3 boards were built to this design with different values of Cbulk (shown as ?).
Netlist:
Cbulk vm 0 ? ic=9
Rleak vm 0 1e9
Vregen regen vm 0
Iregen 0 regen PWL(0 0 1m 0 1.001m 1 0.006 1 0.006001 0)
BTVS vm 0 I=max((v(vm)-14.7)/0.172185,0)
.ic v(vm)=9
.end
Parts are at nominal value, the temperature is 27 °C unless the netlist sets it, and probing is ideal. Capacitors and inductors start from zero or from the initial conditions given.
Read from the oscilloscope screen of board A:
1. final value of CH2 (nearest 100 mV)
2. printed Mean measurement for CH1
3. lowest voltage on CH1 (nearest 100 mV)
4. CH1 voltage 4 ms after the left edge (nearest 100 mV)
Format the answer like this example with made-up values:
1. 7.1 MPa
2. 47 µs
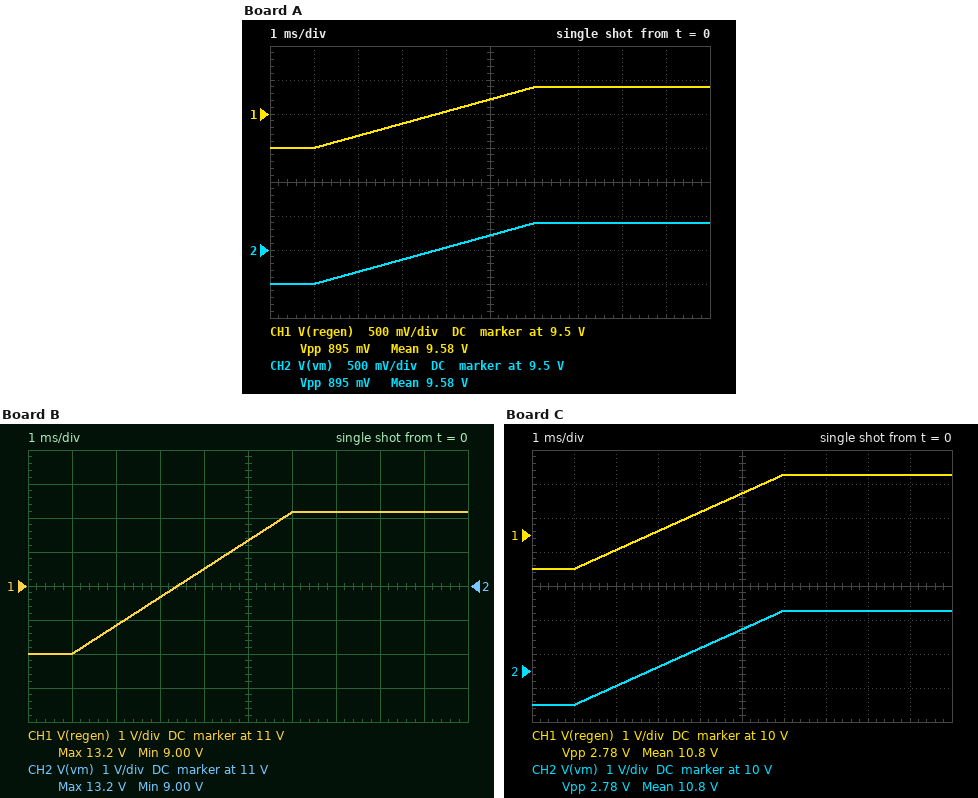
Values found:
1. 9.9 V
2. 9.58 V
3. 9.0 V
4. 9.5 V
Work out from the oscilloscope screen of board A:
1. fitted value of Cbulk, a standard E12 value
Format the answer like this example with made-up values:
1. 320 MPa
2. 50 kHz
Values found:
1. 5.6 mF
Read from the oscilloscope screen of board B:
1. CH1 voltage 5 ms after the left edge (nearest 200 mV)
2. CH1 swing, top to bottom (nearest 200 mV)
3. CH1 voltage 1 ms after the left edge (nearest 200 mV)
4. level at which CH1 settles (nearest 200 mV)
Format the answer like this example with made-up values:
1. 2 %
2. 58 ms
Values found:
1. 12.4 V
2. 4.2 V
3. 9.0 V
4. 13.2 V
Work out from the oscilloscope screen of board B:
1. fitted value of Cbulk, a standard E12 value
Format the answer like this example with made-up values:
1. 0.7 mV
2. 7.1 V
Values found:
1. 1.2 mF
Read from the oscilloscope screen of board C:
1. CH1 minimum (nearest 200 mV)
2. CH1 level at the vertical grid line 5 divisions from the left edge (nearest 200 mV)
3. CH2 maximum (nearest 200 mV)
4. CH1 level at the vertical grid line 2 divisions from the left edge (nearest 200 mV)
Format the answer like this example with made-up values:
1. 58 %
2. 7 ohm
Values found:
1. 9.0 V
2. 11.2 V
3. 11.8 V
4. 9.6 V
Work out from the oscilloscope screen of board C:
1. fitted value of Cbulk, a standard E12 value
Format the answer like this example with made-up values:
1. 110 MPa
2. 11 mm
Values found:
1. 1.8 mF
